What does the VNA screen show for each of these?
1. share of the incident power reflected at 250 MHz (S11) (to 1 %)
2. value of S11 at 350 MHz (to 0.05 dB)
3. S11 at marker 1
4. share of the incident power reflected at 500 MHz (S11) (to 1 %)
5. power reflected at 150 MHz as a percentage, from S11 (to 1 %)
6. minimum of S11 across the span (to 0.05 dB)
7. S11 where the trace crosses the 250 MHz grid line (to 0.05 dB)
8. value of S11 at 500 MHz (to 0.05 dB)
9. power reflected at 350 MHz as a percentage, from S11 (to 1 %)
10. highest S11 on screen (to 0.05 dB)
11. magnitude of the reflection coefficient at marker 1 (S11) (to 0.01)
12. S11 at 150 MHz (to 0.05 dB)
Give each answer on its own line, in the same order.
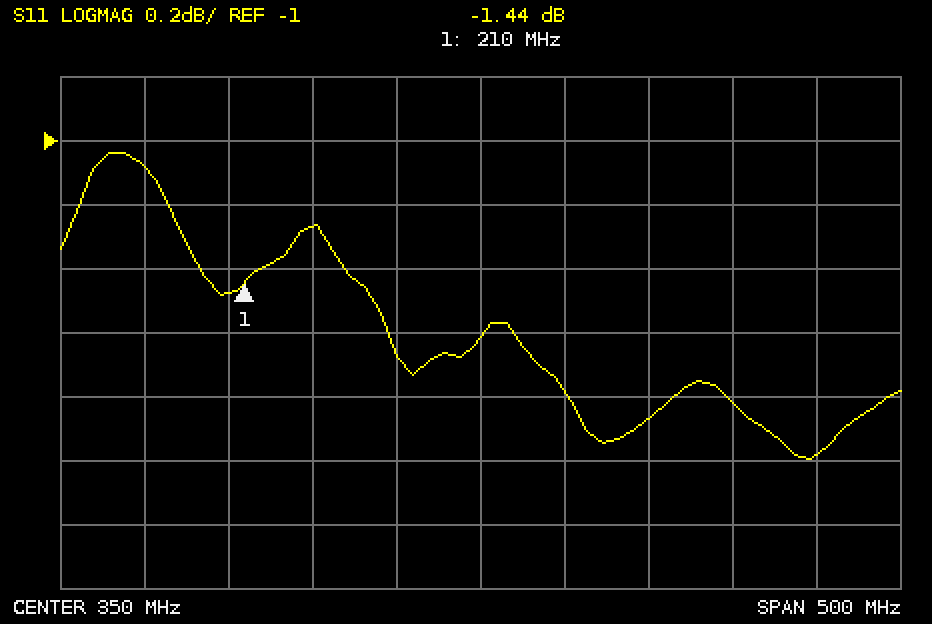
75 %
-1.60 dB
-1.44 dB
66 %
78 %
-2.00 dB
-1.25 dB
-1.80 dB
69 %
-1.05 dB
0.85
-1.10 dB
